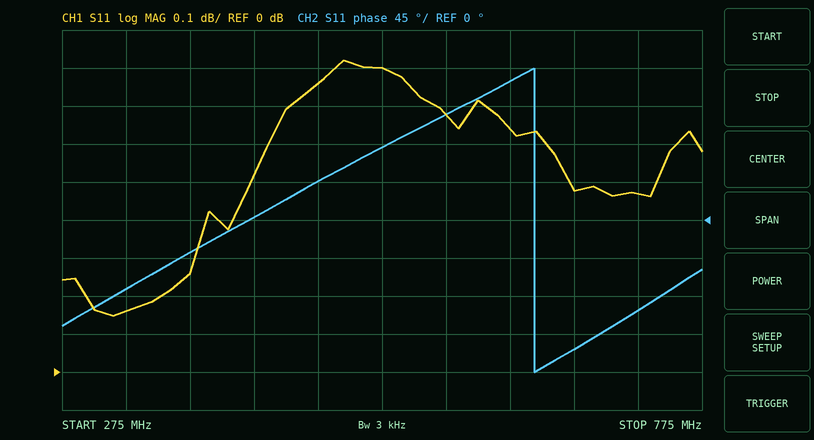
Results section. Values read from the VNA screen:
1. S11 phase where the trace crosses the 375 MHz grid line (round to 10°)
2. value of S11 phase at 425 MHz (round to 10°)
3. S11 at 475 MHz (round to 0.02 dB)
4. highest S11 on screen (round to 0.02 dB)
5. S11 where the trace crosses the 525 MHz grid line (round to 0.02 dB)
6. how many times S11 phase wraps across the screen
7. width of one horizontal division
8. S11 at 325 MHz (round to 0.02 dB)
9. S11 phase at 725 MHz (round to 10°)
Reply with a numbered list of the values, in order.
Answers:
1. -40°
2. 0°
3. 0.76 dB
4. 0.82 dB
5. 0.80 dB
6. 1
7. 50 MHz
8. 0.16 dB
9. -110°
